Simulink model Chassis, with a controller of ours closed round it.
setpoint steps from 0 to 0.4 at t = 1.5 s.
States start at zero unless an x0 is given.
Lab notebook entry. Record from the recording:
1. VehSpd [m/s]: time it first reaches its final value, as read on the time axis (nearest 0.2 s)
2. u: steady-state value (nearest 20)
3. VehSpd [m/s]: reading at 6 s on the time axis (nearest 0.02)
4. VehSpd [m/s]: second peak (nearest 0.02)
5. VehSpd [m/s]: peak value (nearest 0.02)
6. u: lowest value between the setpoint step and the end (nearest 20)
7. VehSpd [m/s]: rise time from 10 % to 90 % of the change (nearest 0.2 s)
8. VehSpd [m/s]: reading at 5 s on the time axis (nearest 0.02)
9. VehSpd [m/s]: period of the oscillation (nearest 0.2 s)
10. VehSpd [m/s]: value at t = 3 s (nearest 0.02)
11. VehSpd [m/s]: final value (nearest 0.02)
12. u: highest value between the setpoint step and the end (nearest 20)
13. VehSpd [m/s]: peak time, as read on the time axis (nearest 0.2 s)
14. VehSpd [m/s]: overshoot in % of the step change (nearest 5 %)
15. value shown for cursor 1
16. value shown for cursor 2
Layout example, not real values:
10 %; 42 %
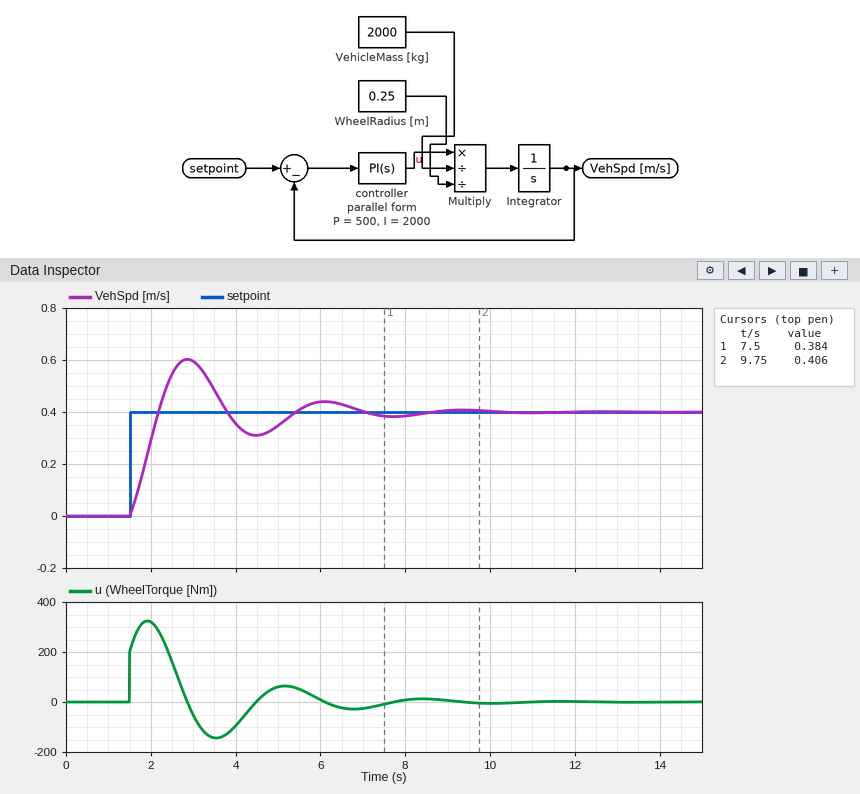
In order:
2.2 s; 0; 0.44; 0.44; 0.60; -140; 0.6 s; 0.34; 3.2 s; 0.60; 0.40; 320; 2.8 s; 50 %; 0.384; 0.406
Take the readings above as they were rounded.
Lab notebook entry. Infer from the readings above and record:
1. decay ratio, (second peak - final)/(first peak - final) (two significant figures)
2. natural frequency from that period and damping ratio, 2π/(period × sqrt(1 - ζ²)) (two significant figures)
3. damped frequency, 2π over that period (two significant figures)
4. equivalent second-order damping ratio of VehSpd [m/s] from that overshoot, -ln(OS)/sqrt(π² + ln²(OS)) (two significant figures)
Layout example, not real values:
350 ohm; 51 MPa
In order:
0.20; 2.0 rad/s; 2.0 rad/s; 0.22
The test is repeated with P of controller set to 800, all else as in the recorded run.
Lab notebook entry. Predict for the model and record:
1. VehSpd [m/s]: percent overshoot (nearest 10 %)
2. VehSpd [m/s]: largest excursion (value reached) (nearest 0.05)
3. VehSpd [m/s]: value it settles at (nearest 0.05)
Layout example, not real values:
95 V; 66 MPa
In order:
40 %; 0.55; 0.40
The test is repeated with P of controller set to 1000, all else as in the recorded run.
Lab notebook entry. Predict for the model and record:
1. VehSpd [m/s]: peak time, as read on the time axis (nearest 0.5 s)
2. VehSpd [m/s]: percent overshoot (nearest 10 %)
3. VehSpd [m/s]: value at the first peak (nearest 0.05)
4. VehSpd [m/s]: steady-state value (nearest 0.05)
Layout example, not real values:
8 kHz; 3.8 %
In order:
2.5 s; 30 %; 0.50; 0.40
